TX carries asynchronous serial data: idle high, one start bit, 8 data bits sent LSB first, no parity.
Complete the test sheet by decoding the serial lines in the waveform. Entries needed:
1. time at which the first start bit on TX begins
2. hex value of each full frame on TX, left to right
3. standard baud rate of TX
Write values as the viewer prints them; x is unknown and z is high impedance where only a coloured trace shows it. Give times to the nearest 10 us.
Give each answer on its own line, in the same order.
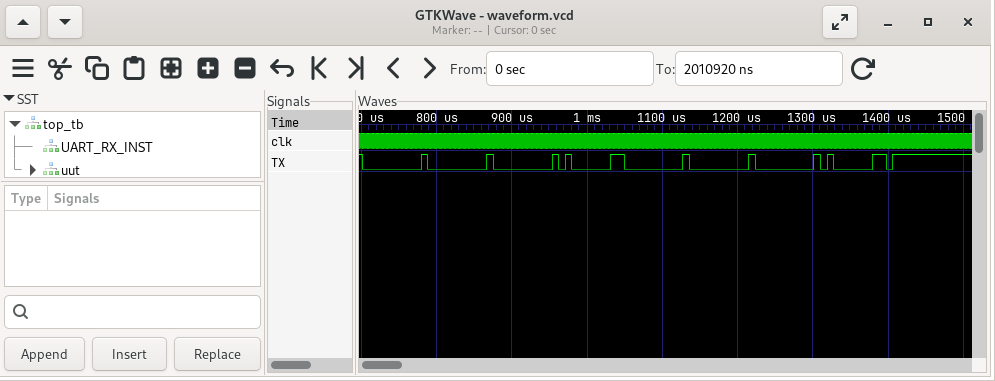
700 us
00, 00, 00, 81, 00, 00, 00, 81, FF
115200 baud
